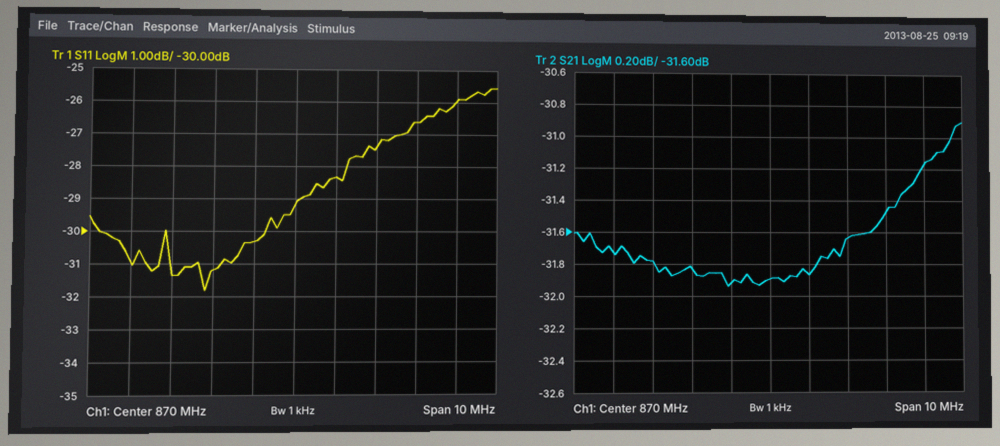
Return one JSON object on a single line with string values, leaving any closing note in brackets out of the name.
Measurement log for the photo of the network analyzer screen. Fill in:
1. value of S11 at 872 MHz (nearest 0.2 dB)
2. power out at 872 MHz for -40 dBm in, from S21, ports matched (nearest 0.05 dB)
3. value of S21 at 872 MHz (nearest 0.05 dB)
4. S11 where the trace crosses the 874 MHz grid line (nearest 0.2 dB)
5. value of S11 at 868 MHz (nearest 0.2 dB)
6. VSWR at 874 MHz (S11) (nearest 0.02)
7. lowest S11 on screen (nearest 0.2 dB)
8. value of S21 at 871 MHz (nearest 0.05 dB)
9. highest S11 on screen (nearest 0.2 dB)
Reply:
{"value of S11 at 872 MHz": "-27.4 dB", "power out at 872 MHz for -40 dBm in, from S21, ports matched": "-71.65 dBm", "value of S21 at 872 MHz": "-31.65 dB", "S11 where the trace crosses the 874 MHz grid line": "-26.0 dB", "value of S11 at 868 MHz": "-31.2 dB", "VSWR at 874 MHz (S11)": "1.10", "lowest S11 on screen": "-31.8 dB", "value of S21 at 871 MHz": "-31.85 dB", "highest S11 on screen": "-25.6 dB"}
